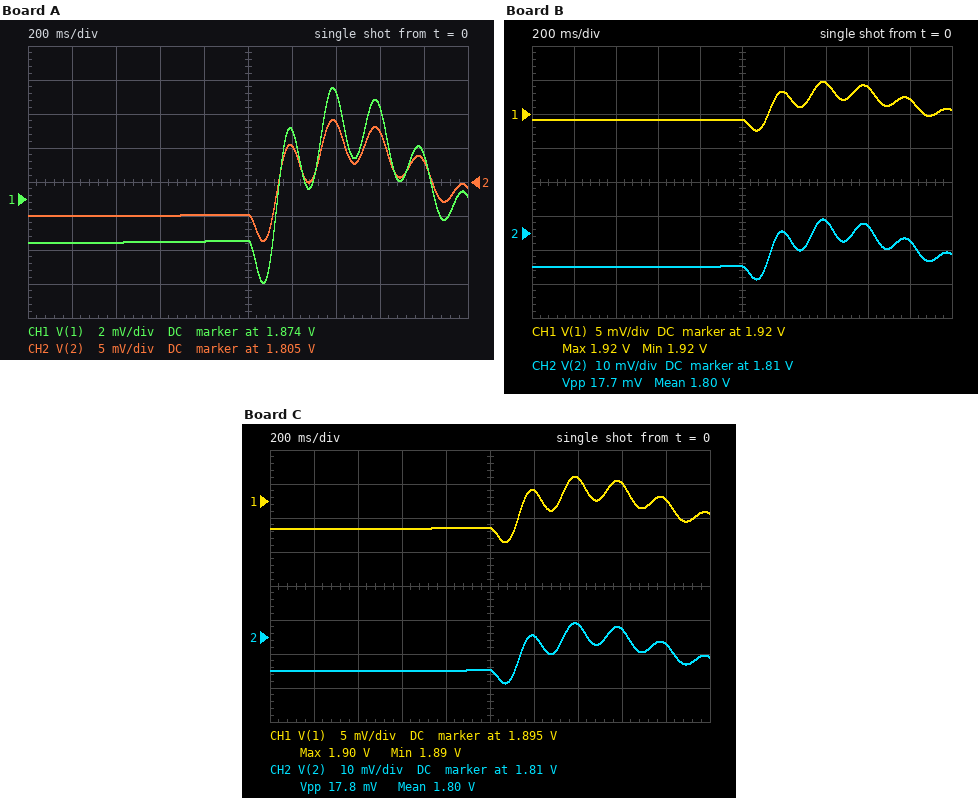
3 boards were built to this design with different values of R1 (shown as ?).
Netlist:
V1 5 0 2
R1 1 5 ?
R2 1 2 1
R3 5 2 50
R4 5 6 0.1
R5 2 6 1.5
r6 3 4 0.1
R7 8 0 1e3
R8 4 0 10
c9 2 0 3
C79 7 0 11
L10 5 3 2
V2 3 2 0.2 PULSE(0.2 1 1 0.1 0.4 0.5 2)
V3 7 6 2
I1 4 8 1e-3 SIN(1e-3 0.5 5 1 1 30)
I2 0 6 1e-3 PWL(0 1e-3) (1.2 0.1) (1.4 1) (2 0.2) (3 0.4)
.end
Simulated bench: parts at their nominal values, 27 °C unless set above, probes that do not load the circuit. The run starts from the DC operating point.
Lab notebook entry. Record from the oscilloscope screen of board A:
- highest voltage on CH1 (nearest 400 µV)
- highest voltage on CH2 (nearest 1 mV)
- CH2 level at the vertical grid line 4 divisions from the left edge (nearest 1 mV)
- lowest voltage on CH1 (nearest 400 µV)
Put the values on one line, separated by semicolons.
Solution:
1.8804 V; 1.814 V; 1.800 V; 1.8692 V
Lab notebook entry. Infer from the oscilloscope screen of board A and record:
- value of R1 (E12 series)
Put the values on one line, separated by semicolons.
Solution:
1.8 Ω
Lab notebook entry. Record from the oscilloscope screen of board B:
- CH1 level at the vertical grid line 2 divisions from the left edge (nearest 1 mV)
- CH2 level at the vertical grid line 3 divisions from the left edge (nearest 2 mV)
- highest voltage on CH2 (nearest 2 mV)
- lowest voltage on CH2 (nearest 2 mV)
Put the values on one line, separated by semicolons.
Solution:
1.919 V; 1.800 V; 1.814 V; 1.796 V
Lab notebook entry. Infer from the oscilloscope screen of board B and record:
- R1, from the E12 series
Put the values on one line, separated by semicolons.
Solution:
0.68 Ω
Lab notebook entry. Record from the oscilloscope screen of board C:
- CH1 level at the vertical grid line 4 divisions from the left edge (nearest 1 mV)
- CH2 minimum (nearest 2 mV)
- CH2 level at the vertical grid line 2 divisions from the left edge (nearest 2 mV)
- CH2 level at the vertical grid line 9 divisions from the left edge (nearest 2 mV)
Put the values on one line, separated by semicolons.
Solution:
1.891 V; 1.796 V; 1.800 V; 1.808 V
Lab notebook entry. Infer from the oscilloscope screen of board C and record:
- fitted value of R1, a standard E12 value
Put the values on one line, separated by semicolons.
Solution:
1.2 Ω
